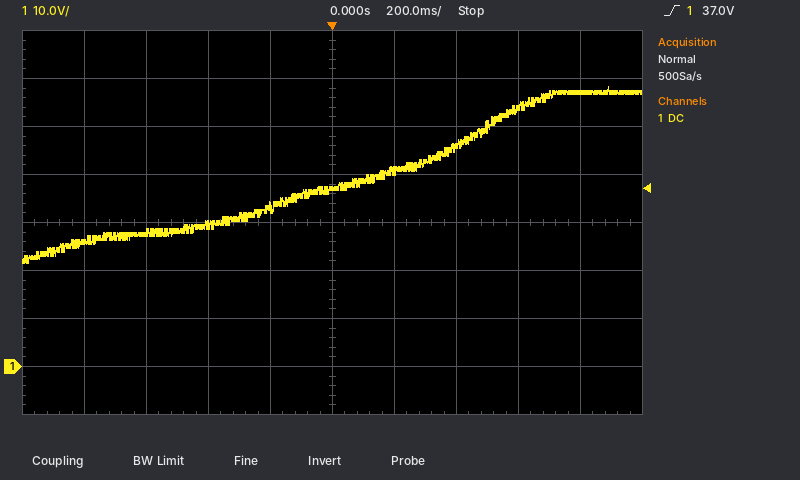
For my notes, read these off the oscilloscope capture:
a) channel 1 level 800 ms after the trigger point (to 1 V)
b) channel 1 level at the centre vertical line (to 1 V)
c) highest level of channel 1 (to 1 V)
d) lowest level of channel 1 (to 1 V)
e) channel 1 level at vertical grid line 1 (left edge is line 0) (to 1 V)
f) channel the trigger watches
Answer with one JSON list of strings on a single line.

["57 V", "37 V", "58 V", "22 V", "26 V", "channel 1"]
